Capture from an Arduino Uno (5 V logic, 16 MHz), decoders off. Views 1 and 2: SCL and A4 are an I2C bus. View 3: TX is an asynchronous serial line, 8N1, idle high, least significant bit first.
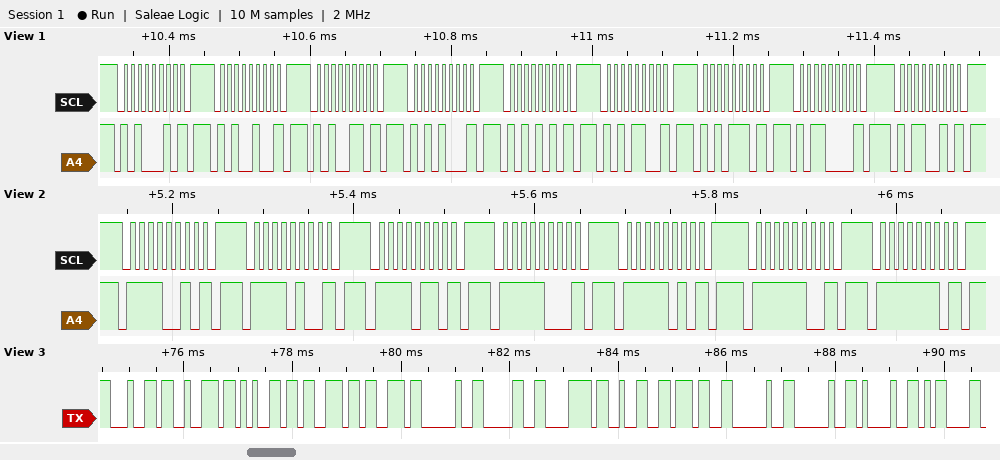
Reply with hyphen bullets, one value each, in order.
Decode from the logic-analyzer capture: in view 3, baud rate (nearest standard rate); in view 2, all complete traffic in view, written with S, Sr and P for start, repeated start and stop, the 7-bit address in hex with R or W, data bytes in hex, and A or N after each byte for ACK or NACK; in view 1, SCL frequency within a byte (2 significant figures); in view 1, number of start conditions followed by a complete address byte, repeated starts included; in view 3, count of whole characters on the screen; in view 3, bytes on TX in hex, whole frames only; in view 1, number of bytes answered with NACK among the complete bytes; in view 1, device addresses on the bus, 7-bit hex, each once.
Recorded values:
- 9600 baud
- S 79W N P S 7AW N P S 7BW N P S 7CW N P S 7DW N P S 7EW N P S 7FW N P
- 100 kHz
- 9
- 14
- 0x64 0x72 0x65 0x73 0x73 0x20 0x30 0x78 0x32 0x37 0x20 0x20 0x21 0x0D
- 9
- 0x51 0x52 0x53 0x54 0x55 0x56 0x57 0x58 0x59
